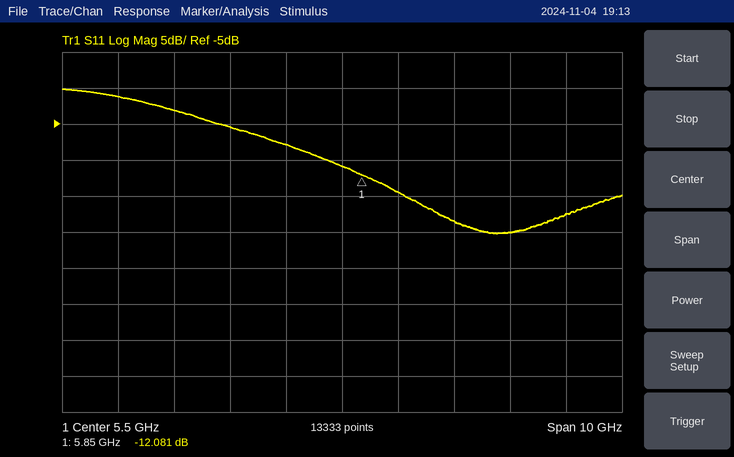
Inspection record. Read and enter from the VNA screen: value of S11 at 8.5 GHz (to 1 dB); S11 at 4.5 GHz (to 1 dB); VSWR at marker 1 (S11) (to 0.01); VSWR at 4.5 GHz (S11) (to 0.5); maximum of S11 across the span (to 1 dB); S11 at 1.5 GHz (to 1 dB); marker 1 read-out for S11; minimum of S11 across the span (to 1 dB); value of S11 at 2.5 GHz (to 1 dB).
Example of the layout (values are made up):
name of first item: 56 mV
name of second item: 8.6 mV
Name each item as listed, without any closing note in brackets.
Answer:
value of S11 at 8.5 GHz: -20 dB
S11 at 4.5 GHz: -8 dB
VSWR at marker 1 (S11): 1.66
VSWR at 4.5 GHz (S11): 2.5
maximum of S11 across the span: 0 dB
S11 at 1.5 GHz: -1 dB
marker 1 read-out for S11: -12.081 dB
minimum of S11 across the span: -20 dB
value of S11 at 2.5 GHz: -3 dB
